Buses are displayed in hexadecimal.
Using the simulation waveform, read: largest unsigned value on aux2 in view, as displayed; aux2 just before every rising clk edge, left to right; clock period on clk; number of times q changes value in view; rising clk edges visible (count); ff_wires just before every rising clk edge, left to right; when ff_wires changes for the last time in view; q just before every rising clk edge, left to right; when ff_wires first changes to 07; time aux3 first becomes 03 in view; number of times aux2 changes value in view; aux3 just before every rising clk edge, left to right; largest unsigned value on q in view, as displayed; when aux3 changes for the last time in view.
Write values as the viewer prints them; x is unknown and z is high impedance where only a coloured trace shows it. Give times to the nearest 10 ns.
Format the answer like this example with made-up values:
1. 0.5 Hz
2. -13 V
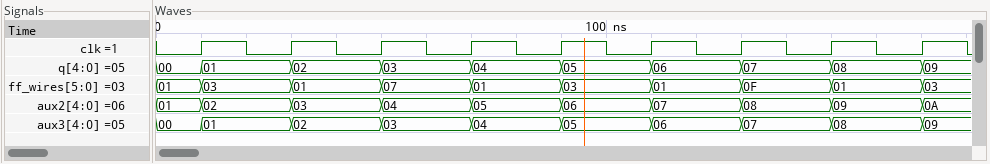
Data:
1. 0A
2. 01, 02, 03, 04, 05, 06, 07, 08, 09
3. 20 ns
4. 9
5. 9
6. 01, 03, 01, 07, 01, 03, 01, 0F, 01
7. 170 ns
8. 00, 01, 02, 03, 04, 05, 06, 07, 08
9. 50 ns
10. 50 ns
11. 9
12. 00, 01, 02, 03, 04, 05, 06, 07, 08
13. 09
14. 170 ns
